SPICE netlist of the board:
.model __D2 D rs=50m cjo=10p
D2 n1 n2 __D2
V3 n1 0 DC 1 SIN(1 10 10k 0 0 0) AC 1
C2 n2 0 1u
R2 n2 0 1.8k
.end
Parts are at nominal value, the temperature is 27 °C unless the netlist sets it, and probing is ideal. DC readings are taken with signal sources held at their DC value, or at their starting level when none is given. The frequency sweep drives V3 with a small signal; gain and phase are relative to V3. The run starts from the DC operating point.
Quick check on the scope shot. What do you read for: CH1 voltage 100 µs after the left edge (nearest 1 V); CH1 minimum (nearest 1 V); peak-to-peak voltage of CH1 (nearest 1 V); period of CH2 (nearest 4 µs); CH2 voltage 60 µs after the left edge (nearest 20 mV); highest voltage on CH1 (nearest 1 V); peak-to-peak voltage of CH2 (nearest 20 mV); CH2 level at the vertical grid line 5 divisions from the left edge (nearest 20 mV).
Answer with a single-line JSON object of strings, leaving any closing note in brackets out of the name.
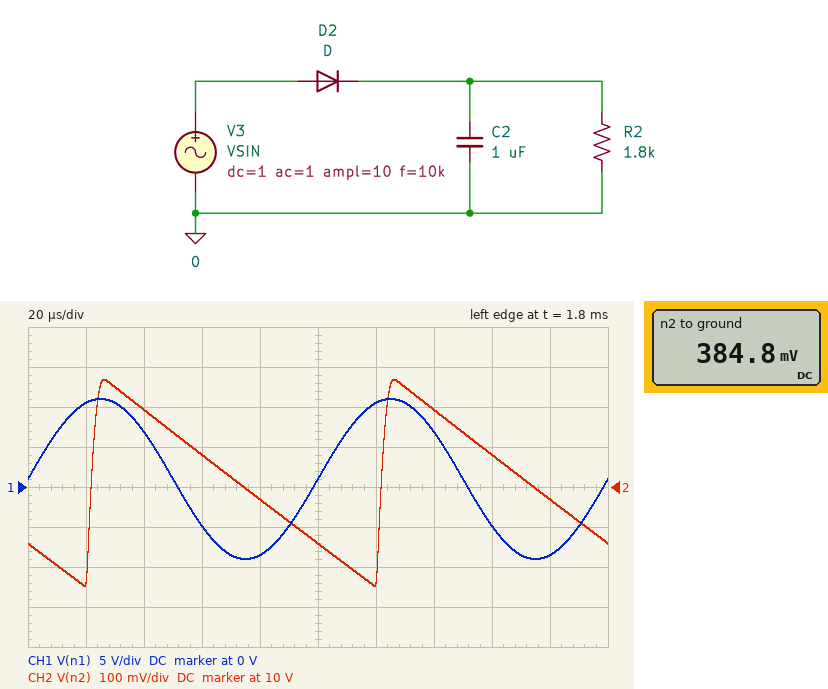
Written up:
{"CH1 voltage 100 µs after the left edge": "1 V", "CH1 minimum": "-9 V", "peak-to-peak voltage of CH1": "20 V", "period of CH2": "100 µs", "CH2 voltage 60 µs after the left edge": "10.08 V", "highest voltage on CH1": "11 V", "peak-to-peak voltage of CH2": "520 mV", "CH2 level at the vertical grid line 5 divisions from the left edge": "9.86 V"}
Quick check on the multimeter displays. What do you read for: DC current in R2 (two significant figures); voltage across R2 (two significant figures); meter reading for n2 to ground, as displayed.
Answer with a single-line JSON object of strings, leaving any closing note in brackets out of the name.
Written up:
{"DC current in R2": "210 µA", "voltage across R2": "380 mV", "meter reading for n2 to ground, as displayed": "384.8 mV"}
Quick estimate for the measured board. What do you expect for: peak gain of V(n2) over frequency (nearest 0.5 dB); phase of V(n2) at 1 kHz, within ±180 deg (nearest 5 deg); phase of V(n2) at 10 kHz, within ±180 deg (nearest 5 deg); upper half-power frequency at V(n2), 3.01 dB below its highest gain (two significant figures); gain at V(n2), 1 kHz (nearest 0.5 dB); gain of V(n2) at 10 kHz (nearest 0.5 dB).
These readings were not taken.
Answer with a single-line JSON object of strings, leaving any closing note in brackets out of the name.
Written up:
{"peak gain of V(n2) over frequency": "-0.5 dB", "phase of V(n2) at 1 kHz, within ±180 deg": "-35 deg", "phase of V(n2) at 10 kHz, within ±180 deg": "-80 deg", "upper half-power frequency at V(n2), 3.01 dB below its highest gain": "1.4 kHz", "gain at V(n2), 1 kHz": "-2.5 dB", "gain of V(n2) at 10 kHz": "-17.5 dB"}
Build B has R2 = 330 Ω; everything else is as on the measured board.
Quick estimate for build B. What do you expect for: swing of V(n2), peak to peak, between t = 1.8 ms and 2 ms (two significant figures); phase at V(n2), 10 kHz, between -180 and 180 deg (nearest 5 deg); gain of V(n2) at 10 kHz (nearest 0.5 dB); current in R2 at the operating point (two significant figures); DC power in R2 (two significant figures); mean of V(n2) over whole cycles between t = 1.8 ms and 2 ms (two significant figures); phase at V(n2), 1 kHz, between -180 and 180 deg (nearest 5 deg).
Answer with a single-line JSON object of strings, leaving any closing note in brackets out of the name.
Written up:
{"swing of V(n2), peak to peak, between t = 1.8 ms and 2 ms": "2.4 V", "phase at V(n2), 10 kHz, between -180 and 180 deg": "-55 deg", "gain of V(n2) at 10 kHz": "-5.5 dB", "current in R2 at the operating point": "1.0 mA", "DC power in R2": "360 µW", "mean of V(n2) over whole cycles between t = 1.8 ms and 2 ms": "9.1 V", "phase at V(n2), 1 kHz, between -180 and 180 deg": "-10 deg"}
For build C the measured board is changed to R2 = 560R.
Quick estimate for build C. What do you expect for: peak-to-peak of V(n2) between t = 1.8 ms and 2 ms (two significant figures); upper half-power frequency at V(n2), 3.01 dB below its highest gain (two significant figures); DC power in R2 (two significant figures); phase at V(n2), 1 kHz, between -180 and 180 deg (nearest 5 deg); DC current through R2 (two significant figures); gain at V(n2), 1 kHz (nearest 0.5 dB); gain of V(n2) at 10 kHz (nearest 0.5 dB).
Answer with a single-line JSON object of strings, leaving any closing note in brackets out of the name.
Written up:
{"peak-to-peak of V(n2) between t = 1.8 ms and 2 ms": "1.5 V", "upper half-power frequency at V(n2), 3.01 dB below its highest gain": "4.2 kHz", "DC power in R2": "230 µW", "phase at V(n2), 1 kHz, between -180 and 180 deg": "-15 deg", "DC current through R2": "640 µA", "gain at V(n2), 1 kHz": "-1.0 dB", "gain of V(n2) at 10 kHz": "-9.0 dB"}
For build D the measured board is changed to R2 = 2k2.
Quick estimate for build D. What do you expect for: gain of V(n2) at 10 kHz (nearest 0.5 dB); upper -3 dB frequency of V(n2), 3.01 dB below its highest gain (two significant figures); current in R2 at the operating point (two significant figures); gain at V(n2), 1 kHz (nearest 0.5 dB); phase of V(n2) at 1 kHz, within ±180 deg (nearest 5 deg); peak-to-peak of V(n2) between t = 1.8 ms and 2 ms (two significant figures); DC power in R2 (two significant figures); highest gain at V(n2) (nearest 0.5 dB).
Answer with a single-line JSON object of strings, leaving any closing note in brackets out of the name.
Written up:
{"gain of V(n2) at 10 kHz": "-19.5 dB", "upper -3 dB frequency of V(n2), 3.01 dB below its highest gain": "1.2 kHz", "current in R2 at the operating point": "180 µA", "gain at V(n2), 1 kHz": "-3.0 dB", "phase of V(n2) at 1 kHz, within ±180 deg": "-40 deg", "peak-to-peak of V(n2) between t = 1.8 ms and 2 ms": "430 mV", "DC power in R2": "69 µW", "highest gain at V(n2)": "-0.5 dB"}
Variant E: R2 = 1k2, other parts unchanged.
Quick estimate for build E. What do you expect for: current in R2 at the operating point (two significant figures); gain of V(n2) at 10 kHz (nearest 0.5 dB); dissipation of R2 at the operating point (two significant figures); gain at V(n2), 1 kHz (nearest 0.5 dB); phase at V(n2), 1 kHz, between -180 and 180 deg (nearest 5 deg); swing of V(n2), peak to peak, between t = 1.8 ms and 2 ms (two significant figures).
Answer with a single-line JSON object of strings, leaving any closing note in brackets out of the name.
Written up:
{"current in R2 at the operating point": "310 µA", "gain of V(n2) at 10 kHz": "-14.5 dB", "dissipation of R2 at the operating point": "120 µW", "gain at V(n2), 1 kHz": "-1.5 dB", "phase at V(n2), 1 kHz, between -180 and 180 deg": "-25 deg", "swing of V(n2), peak to peak, between t = 1.8 ms and 2 ms": "760 mV"}
